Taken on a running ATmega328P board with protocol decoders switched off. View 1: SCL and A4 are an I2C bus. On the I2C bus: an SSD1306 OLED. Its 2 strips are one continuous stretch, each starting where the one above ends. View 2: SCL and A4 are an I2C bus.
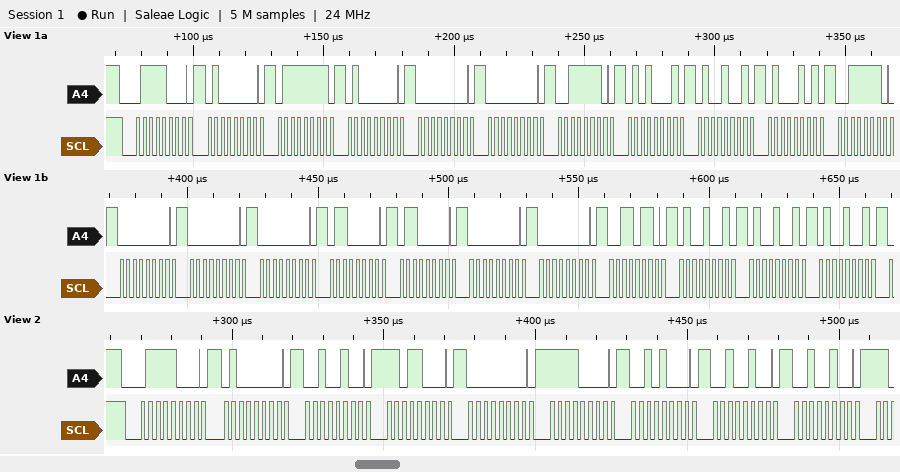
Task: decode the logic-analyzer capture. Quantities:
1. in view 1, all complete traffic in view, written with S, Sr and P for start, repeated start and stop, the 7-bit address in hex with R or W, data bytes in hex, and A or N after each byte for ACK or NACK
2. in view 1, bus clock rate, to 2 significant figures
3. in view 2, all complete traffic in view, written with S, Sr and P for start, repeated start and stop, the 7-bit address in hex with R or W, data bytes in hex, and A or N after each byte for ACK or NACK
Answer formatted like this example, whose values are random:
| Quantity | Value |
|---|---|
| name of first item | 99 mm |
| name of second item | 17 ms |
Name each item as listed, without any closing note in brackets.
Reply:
| Quantity | Value |
|---|---|
| in view 1, all complete traffic in view, written with S, Sr and P for start, repeated start and stop, the 7-bit address in hex with R or W, data bytes in hex, and A or N after each byte for ACK or NACK | S 3CW A 40 A 7F A 40 A 00 A 00 A 3E A 51 A 49 A 45 A 3E A 00 A 00 A 00 A 60 A 60 A 00 A 00 A 36 A 49 A 49 A 49 A |
| in view 1, bus clock rate, to 2 significant figures | 400 kHz |
| in view 2, all complete traffic in view, written with S, Sr and P for start, repeated start and stop, the 7-bit address in hex with R or W, data bytes in hex, and A or N after each byte for ACK or NACK | S 3CW A 40 A 24 A D8 A 00 A F0 A 28 A 24 A 24 A |
